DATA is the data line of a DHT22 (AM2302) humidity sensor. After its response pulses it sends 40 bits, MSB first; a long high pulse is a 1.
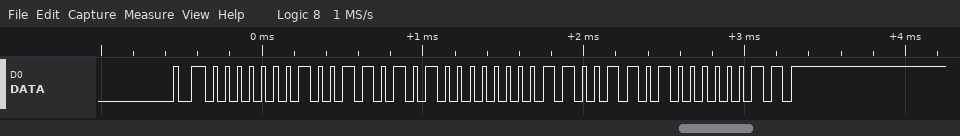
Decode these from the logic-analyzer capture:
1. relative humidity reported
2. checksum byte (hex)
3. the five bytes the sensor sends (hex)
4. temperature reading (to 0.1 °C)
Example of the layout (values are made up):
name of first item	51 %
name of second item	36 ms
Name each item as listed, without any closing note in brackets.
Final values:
relative humidity reported	30.9 %
checksum byte	0x03
the five bytes the sensor sends	01 35 00 CD 03
temperature reading	20.5 °C
